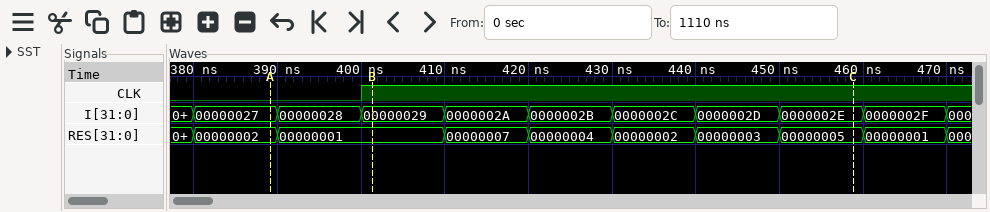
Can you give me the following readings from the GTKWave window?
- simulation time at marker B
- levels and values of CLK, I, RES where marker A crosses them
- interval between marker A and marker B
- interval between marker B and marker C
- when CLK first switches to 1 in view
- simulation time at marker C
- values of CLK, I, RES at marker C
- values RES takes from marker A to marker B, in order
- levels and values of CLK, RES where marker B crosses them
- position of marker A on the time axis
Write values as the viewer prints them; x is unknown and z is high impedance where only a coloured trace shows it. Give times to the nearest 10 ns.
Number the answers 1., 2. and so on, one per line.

1. 400 ns
2. CLK=0, I=00000027, RES=00000002
3. 10 ns
4. 60 ns
5. 400 ns
6. 460 ns
7. CLK=1, I=0000002E, RES=00000005
8. 00000002, 00000001
9. CLK=1, RES=00000001
10. 390 ns
